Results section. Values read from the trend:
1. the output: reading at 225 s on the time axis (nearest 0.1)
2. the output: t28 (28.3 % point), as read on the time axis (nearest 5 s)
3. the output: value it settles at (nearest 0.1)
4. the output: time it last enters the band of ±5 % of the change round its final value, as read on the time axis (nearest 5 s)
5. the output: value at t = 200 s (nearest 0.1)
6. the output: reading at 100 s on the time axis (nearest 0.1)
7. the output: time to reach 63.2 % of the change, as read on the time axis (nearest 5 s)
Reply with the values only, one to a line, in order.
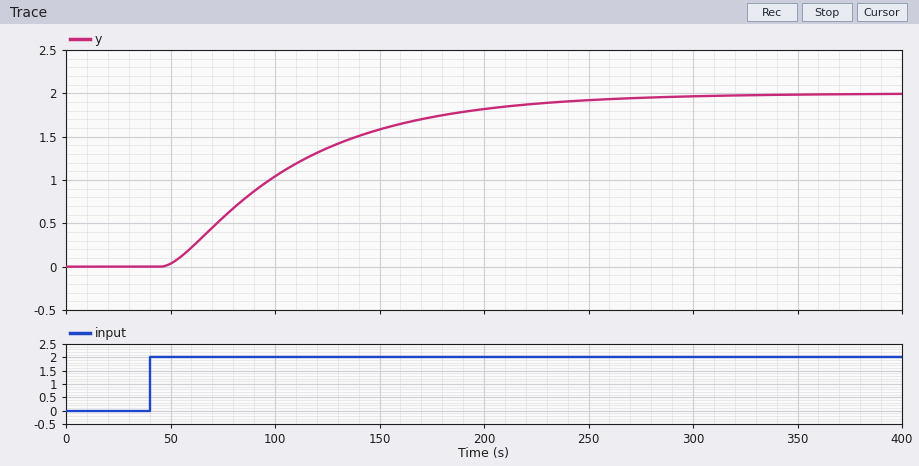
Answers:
1.9
75 s
2.0
235 s
1.8
1.0
115 s
